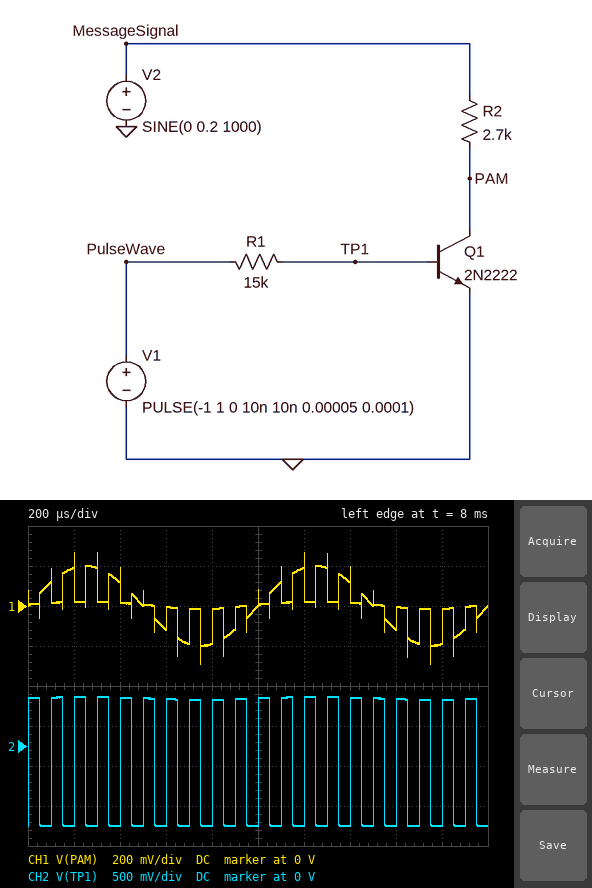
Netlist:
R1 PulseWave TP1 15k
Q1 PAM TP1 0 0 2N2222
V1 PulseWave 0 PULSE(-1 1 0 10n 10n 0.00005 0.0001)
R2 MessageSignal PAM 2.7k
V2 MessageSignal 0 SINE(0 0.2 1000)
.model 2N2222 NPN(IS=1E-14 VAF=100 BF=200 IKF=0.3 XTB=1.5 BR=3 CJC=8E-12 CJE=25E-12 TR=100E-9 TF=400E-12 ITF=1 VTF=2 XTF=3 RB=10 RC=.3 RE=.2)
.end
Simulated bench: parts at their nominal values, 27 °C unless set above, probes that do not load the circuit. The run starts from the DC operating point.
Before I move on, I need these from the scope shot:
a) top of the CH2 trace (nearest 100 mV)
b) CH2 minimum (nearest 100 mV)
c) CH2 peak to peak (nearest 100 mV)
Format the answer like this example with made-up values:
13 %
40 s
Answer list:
600 mV
-1.0 V
1.6 V
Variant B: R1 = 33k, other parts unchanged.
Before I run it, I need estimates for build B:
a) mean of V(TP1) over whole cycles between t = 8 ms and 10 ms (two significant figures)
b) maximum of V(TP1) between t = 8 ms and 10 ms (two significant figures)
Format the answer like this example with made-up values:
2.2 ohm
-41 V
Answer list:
-210 mV
600 mV
